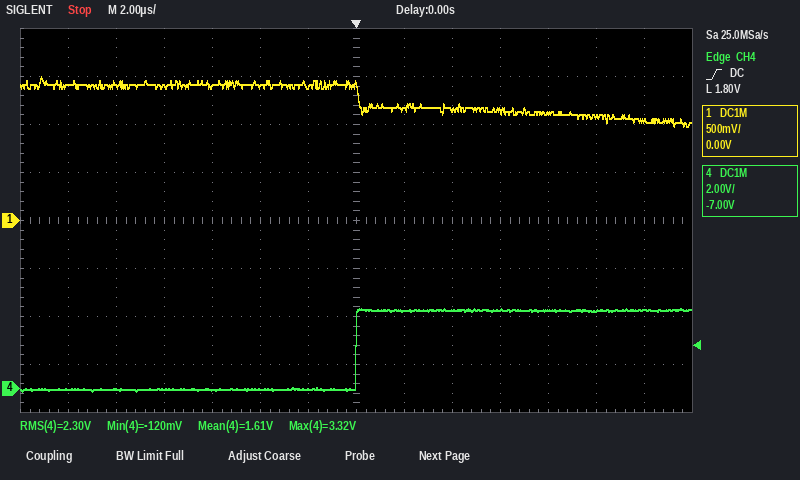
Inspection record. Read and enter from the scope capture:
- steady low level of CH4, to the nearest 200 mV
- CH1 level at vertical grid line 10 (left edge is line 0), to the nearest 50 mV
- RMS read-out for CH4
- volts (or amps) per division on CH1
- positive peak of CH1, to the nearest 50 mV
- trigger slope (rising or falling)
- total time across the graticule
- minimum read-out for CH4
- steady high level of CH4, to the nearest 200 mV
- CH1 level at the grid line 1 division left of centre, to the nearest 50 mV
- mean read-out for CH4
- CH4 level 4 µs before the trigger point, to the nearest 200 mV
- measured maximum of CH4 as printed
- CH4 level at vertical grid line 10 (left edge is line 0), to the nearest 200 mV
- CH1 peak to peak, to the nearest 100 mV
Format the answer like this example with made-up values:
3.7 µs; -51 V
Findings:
0.0 V; 1.15 V; 2.30 V; 500 mV; 1.50 V; rising; 28 µs; -120 mV; 3.2 V; 1.40 V; 1.61 V; 0.0 V; 3.32 V; 3.2 V; 500 mV
